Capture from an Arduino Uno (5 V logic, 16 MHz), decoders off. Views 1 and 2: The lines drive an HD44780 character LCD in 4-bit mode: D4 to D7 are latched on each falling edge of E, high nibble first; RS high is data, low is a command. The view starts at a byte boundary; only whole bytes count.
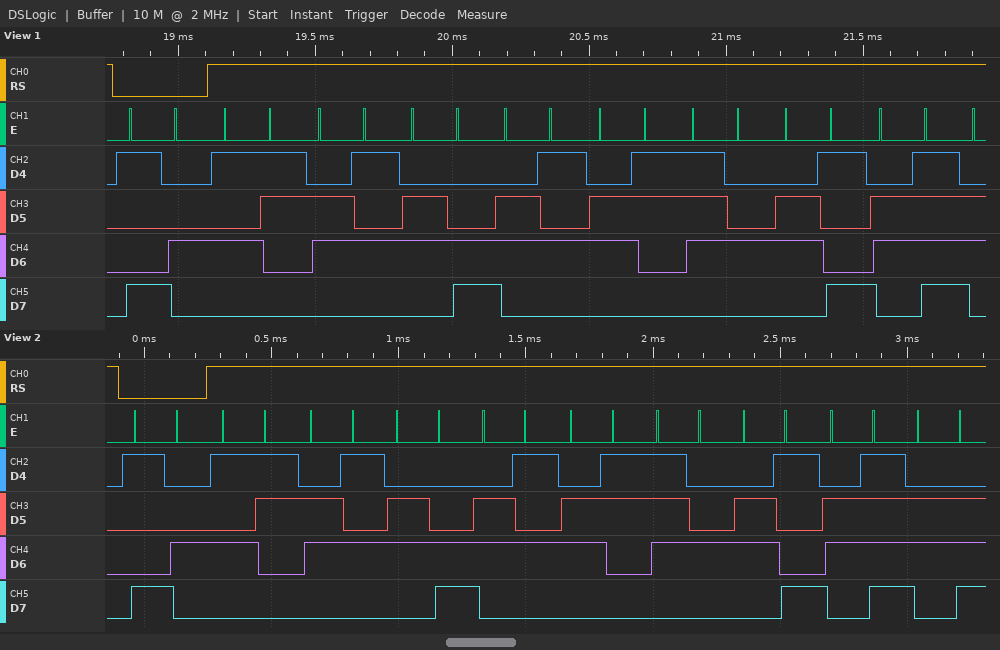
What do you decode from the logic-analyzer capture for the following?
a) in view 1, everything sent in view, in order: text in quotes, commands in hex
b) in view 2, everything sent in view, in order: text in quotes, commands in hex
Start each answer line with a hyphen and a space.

- 0x94 "Selectio"
- 0x94 "Selection"
